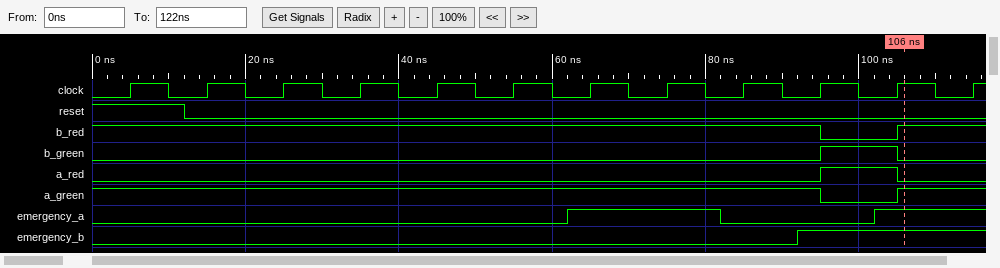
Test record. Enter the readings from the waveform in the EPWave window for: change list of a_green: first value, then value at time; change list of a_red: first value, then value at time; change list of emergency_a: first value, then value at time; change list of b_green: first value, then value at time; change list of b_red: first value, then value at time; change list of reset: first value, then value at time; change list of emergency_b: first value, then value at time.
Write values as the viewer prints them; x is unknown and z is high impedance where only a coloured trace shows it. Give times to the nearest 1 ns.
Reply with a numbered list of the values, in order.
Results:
1. 1, 0 at 95 ns, 1 at 105 ns
2. 0, 1 at 95 ns, 0 at 105 ns
3. 0, 1 at 62 ns, 0 at 82 ns, 1 at 102 ns
4. 0, 1 at 95 ns, 0 at 105 ns
5. 1, 0 at 95 ns, 1 at 105 ns
6. 1, 0 at 12 ns
7. 0, 1 at 92 ns
